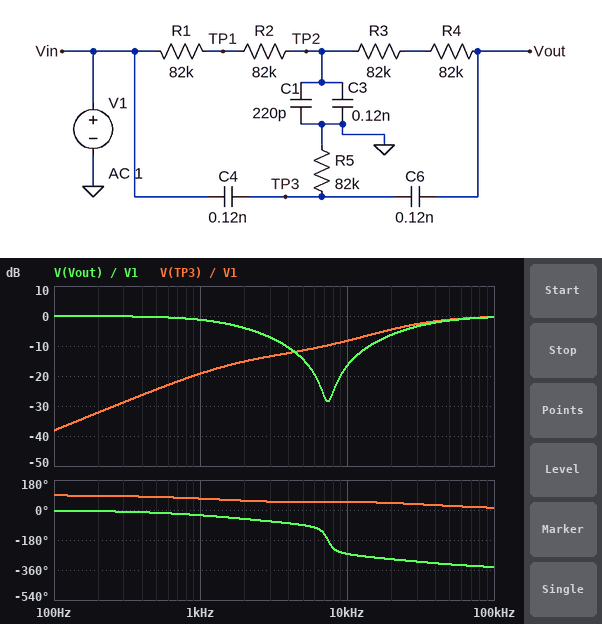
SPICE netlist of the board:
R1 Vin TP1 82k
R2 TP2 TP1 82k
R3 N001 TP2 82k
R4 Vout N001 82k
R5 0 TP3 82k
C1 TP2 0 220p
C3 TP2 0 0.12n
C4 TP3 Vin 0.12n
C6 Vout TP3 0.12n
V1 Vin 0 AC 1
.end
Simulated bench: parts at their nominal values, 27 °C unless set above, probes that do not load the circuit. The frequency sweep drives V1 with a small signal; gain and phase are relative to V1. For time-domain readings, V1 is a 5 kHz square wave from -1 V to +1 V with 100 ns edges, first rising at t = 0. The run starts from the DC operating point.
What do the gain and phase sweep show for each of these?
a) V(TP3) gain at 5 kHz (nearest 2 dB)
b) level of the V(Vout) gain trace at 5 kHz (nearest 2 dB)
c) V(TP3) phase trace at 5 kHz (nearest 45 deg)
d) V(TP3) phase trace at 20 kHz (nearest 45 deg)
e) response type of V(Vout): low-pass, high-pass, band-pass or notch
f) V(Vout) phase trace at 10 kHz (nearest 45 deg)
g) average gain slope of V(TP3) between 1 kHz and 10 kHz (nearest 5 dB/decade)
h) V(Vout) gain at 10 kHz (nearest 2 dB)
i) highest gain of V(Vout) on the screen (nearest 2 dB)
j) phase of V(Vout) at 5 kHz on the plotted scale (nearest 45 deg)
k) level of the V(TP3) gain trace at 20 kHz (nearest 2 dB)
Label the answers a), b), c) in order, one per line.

a) -12 dB
b) -14 dB
c) 45 deg
d) 45 deg
e) notch
f) -270 deg
g) 10 dB/decade
h) -16 dB
i) 0 dB
j) -90 deg
k) -4 dB
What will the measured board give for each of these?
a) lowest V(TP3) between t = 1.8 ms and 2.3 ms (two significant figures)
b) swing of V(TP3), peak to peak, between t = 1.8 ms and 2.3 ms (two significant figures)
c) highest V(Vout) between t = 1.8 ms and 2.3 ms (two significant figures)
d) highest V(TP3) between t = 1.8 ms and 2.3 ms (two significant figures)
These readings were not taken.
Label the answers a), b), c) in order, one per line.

a) -1.9 V
b) 3.8 V
c) 1.5 V
d) 1.9 V
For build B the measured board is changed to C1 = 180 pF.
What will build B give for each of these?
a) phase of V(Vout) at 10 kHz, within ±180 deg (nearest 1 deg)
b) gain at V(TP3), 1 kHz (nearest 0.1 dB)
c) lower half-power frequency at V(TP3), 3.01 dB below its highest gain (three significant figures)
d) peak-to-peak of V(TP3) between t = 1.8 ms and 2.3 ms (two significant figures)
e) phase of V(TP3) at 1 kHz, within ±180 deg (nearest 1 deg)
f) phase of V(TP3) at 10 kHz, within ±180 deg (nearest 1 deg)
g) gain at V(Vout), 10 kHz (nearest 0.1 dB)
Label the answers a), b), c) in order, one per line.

a) 93 deg
b) -19.1 dB
c) 27.8 kHz
d) 3.8 V
e) 69 deg
f) 47 deg
g) -17.5 dB
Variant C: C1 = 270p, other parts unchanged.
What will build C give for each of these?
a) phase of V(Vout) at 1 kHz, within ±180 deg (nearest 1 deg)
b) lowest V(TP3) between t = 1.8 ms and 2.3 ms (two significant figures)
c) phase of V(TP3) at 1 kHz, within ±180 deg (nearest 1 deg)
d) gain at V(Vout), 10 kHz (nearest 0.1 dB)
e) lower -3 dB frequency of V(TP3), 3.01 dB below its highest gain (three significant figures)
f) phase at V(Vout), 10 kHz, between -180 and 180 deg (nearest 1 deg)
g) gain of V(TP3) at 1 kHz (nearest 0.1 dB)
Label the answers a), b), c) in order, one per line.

a) -34 deg
b) -1.9 V
c) 67 deg
d) -15.6 dB
e) 27.5 kHz
f) 98 deg
g) -19.3 dB
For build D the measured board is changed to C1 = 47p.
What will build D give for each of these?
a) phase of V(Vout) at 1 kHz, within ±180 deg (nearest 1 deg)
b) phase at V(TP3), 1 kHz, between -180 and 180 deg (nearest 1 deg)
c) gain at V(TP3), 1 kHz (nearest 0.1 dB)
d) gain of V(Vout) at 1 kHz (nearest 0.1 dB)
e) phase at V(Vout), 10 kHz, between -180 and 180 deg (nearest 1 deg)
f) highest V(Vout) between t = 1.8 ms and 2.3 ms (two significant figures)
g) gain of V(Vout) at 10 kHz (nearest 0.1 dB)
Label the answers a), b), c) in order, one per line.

a) -23 deg
b) 72 deg
c) -18.8 dB
d) -0.8 dB
e) 49 deg
f) 1.4 V
g) -21.4 dB
